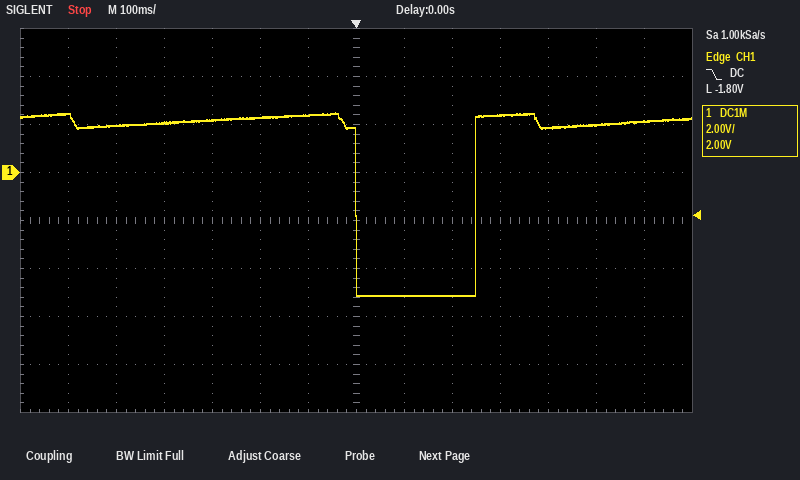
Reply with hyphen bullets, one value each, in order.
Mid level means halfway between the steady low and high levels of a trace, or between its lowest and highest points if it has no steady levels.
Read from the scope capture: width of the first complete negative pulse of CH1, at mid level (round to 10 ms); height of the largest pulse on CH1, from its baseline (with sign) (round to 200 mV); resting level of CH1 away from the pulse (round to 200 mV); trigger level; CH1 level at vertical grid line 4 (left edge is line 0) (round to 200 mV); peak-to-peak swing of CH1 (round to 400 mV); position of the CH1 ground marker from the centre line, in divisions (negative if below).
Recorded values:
- 250 ms
- -7.2 V
- 2.2 V
- -1.80 V
- 2.2 V
- 7.6 V
- +1.0 div
